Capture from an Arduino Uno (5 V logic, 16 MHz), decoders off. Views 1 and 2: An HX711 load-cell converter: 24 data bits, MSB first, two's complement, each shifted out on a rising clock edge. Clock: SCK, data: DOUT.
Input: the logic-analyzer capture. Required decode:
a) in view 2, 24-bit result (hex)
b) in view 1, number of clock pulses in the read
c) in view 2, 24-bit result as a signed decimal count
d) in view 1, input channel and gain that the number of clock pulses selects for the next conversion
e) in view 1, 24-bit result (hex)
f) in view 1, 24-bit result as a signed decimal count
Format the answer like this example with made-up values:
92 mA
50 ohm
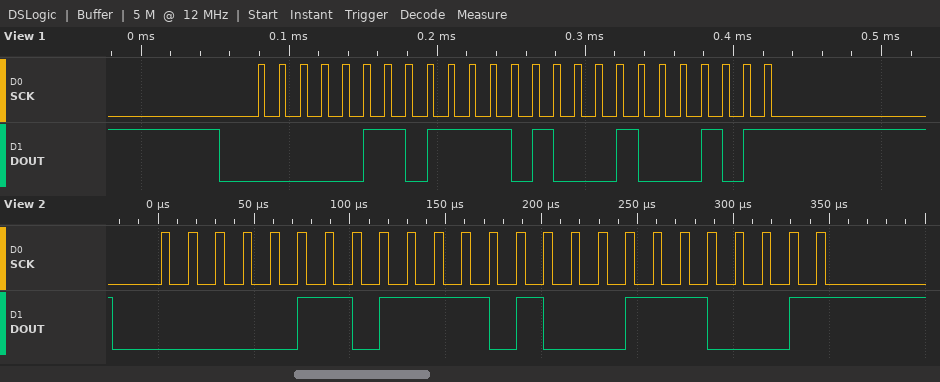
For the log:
0x06F471
25
455793
channel A, gain 128
0x06F445
455749
